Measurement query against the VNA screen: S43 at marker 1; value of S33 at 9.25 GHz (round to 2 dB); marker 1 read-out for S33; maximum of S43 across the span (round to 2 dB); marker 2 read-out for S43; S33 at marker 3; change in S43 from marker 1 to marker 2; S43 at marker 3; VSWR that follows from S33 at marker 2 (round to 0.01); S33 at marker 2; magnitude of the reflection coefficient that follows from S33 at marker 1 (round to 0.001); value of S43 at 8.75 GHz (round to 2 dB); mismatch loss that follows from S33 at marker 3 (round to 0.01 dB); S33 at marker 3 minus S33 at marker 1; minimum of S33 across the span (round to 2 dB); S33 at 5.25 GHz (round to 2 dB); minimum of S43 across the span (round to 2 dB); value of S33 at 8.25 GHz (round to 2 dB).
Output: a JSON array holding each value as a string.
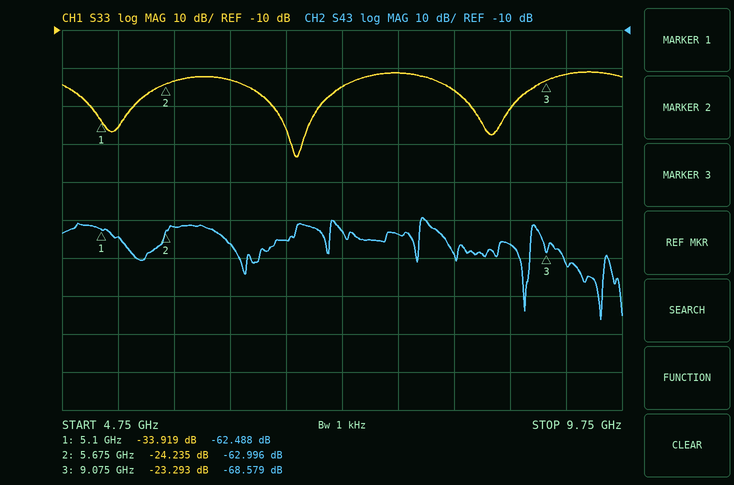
["-62.488 dB", "-22 dB", "-33.919 dB", "-60 dB", "-62.996 dB", "-23.293 dB", "-0.508 dB", "-68.579 dB", "1.13", "-24.235 dB", "0.020", "-66 dB", "0.02 dB", "10.626 dB", "-44 dB", "-36 dB", "-86 dB", "-26 dB"]
